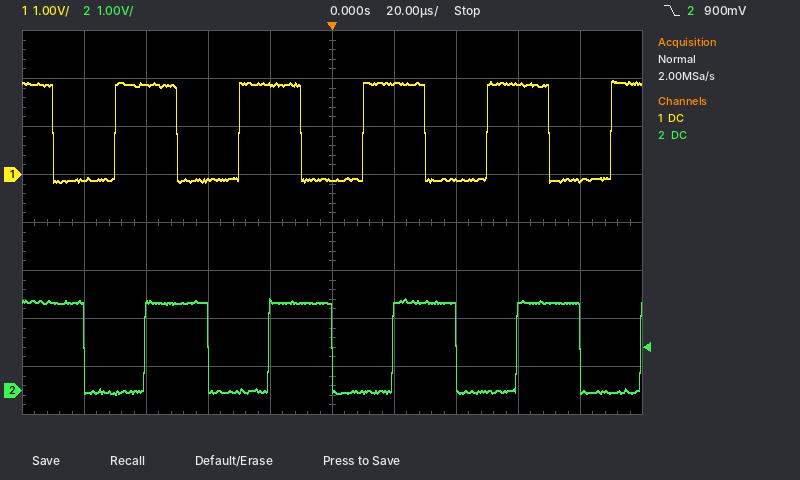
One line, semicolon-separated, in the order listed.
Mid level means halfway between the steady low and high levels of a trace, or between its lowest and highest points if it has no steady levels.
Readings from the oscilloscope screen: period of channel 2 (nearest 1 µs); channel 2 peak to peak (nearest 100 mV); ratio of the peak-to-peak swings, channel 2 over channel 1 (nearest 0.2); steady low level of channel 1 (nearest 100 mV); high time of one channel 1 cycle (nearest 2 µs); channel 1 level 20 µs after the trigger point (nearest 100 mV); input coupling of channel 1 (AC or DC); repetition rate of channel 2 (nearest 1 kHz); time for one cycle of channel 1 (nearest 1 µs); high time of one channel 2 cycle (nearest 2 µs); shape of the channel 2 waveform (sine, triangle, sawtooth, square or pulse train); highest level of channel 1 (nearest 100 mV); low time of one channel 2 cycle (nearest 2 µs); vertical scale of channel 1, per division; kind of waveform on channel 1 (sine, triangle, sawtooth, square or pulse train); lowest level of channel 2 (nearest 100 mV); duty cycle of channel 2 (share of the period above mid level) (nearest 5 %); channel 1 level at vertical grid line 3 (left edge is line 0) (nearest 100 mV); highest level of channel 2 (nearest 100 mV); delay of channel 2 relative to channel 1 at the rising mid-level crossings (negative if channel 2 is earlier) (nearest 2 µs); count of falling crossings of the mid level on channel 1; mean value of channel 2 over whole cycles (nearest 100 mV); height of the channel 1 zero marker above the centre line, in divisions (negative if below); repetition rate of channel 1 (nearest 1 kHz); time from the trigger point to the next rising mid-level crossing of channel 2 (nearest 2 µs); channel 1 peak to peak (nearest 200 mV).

40 µs; 2.0 V; 1.0; -100 mV; 20 µs; 1.9 V; DC; 25 kHz; 40 µs; 20 µs; square; 2.0 V; 20 µs; 1 V; square; -100 mV; 50 %; -100 mV; 1.9 V; +10 µs; 5; 900 mV; +1.0 div; 25 kHz; 20 µs; 2.2 V
